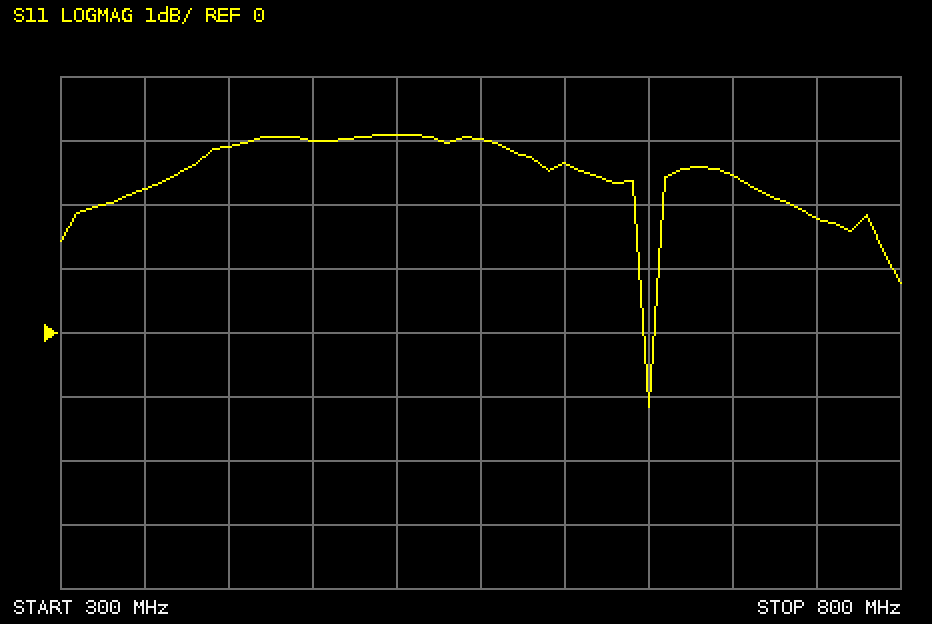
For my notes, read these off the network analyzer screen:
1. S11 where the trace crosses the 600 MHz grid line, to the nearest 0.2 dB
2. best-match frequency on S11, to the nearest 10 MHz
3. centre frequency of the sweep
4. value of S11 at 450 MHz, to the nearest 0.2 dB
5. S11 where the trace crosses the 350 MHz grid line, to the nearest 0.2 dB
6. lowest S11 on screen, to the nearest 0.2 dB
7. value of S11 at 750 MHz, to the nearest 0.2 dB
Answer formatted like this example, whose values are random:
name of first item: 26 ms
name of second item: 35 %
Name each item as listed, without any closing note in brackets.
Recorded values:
S11 where the trace crosses the 600 MHz grid line, to the nearest 0.2 dB: 2.6 dB
best-match frequency on S11, to the nearest 10 MHz: 650 MHz
centre frequency of the sweep: 550 MHz
value of S11 at 450 MHz, to the nearest 0.2 dB: 3.0 dB
S11 where the trace crosses the 350 MHz grid line, to the nearest 0.2 dB: 2.2 dB
lowest S11 on screen, to the nearest 0.2 dB: -1.2 dB
value of S11 at 750 MHz, to the nearest 0.2 dB: 1.8 dB
